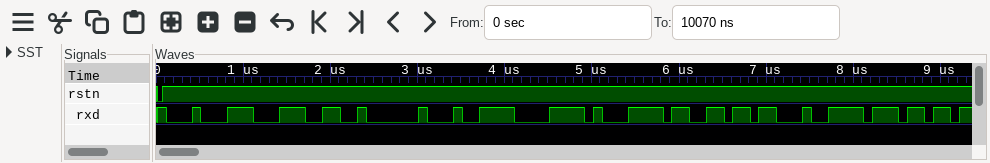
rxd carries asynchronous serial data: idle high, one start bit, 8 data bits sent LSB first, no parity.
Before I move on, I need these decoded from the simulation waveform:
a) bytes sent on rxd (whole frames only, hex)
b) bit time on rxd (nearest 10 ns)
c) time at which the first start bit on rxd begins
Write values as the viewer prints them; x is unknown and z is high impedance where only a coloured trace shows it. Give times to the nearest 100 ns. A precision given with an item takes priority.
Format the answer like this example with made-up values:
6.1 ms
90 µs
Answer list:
C4, 9C, 02, E4, 78, BC, B6, E4, B7
100 ns
100 ns
